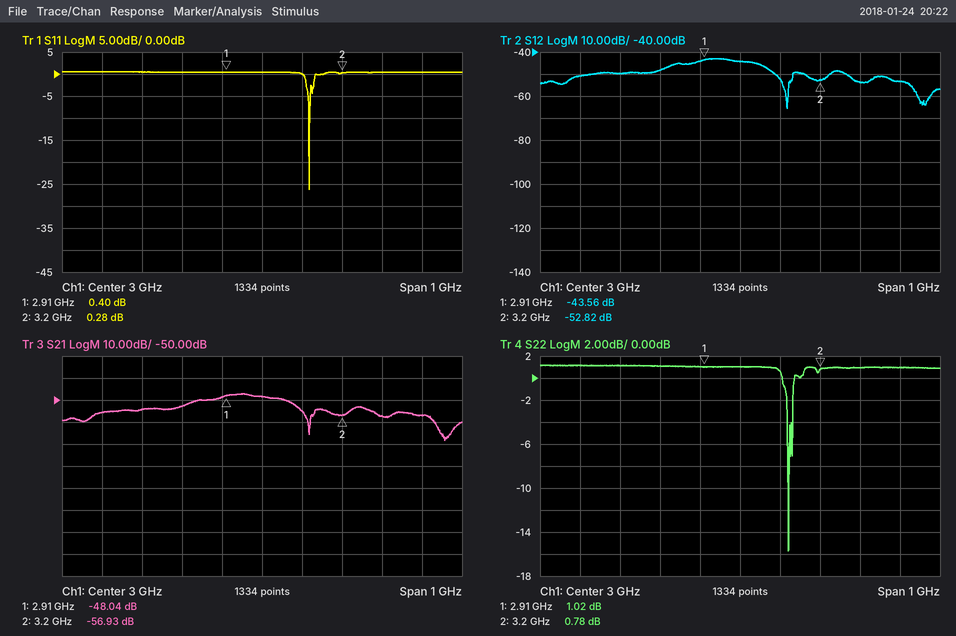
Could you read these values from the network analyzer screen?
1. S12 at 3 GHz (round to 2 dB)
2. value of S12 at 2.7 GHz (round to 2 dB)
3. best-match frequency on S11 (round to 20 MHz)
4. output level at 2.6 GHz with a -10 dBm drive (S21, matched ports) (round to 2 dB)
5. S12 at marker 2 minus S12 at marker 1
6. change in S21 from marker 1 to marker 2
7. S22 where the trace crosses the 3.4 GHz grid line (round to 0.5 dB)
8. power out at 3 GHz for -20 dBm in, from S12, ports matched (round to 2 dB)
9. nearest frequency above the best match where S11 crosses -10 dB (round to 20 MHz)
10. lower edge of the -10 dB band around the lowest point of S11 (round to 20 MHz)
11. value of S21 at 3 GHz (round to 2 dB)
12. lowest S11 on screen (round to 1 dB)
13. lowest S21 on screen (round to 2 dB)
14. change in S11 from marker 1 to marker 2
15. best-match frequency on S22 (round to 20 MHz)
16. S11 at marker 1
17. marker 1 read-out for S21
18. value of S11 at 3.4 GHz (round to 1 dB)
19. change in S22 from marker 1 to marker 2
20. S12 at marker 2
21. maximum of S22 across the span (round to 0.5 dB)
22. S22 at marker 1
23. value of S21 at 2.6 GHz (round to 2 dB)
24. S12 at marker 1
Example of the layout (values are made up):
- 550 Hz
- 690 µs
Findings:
- -44 dB
- -50 dB
- 3.12 GHz
- -66 dBm
- -9.26 dB
- -8.89 dB
- 1.0 dB
- -64 dBm
- 3.12 GHz
- 3.12 GHz
- -48 dB
- -26 dB
- -68 dB
- -0.12 dB
- 3.12 GHz
- 0.40 dB
- -48.04 dB
- 0 dB
- -0.24 dB
- -52.82 dB
- 1.0 dB
- 1.02 dB
- -56 dB
- -43.56 dB
